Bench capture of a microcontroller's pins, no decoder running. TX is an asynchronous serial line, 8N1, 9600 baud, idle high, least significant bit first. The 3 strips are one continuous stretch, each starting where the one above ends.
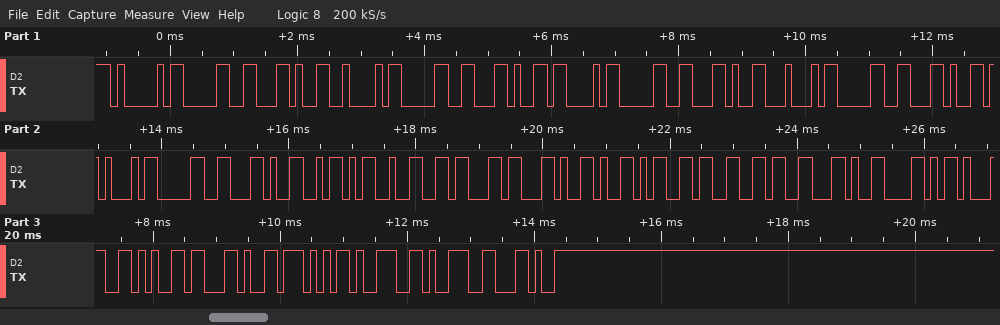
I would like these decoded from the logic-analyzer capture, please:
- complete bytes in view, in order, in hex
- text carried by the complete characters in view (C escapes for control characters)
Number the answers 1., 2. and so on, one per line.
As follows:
1. 41 30 2C 42 30 2C 43 30 2C 44 30 2C 45 30 2C 5A 32 63 2C 59 36 36 2C 58 31 65 2C 57 39 39 2C
2. "A0,B0,C0,D0,E0,Z2c,Y66,X1e,W99,"
